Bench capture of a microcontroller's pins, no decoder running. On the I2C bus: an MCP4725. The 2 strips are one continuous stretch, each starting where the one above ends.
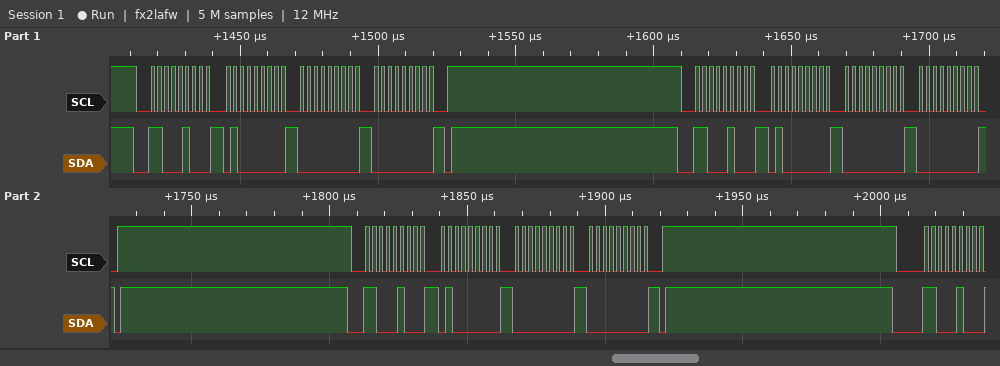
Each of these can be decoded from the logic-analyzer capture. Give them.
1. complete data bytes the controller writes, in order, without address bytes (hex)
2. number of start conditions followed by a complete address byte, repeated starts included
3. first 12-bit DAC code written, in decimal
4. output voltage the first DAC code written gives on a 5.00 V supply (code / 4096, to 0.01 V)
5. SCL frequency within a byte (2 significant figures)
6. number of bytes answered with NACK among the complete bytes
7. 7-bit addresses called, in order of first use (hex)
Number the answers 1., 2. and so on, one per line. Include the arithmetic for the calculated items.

1. 40 00 00 40 00 00 40 00 00
2. 4
3. 0
4. 0 / 4096 x 5.00 V = 0.00 V
5. 400 kHz
6. 0
7. 0x62
